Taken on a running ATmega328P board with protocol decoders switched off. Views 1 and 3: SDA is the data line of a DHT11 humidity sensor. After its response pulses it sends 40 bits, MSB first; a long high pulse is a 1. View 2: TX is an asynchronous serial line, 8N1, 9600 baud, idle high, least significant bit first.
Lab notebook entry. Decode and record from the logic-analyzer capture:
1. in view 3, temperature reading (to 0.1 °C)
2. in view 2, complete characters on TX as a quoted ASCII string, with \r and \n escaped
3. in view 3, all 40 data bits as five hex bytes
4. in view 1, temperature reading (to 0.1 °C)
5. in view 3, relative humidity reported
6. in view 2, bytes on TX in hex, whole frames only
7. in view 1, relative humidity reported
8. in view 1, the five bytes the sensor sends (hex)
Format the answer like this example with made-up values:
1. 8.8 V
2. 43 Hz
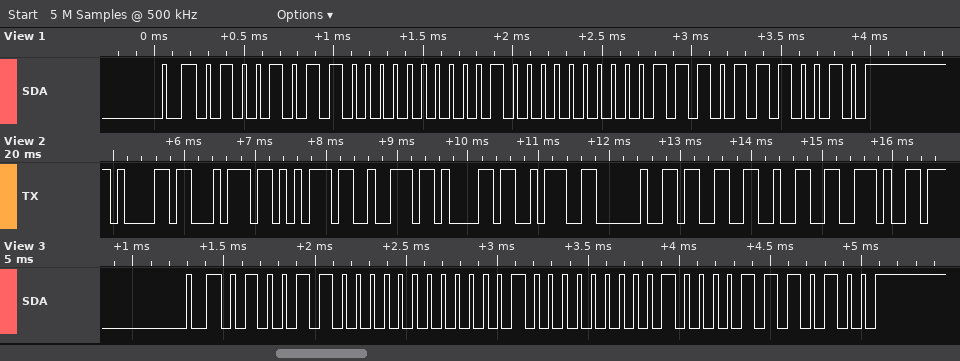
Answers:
1. 32.8 °C
2. "atura: 32."
3. 4C 00 20 08 74
4. 32.7 °C
5. 76 %
6. 0x61 0x74 0x75 0x72 0x61 0x3A 0x20 0x33 0x32 0x2E
7. 75 %
8. 4B 00 20 07 72
